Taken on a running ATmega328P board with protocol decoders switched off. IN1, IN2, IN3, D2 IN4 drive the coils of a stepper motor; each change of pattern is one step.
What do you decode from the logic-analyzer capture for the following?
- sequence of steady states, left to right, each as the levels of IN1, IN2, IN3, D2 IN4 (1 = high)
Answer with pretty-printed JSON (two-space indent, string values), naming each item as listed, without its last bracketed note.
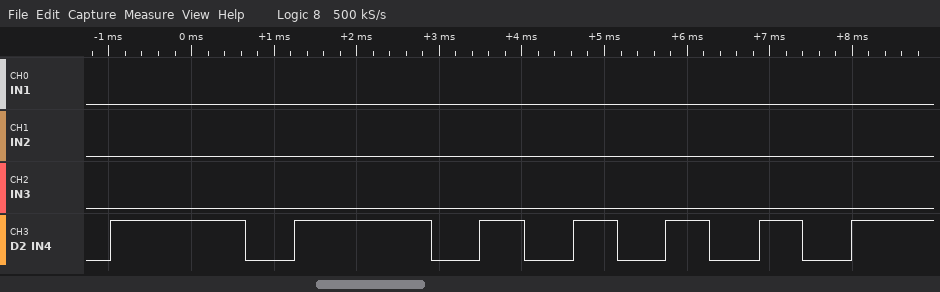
{
  "sequence of steady states, left to right, each as the levels of IN1, IN2, IN3, D2 IN4": "0000 0001 0000 0001 0000 0001 0000 0001 0000 0001 0000 0001 0000 0001"
}
